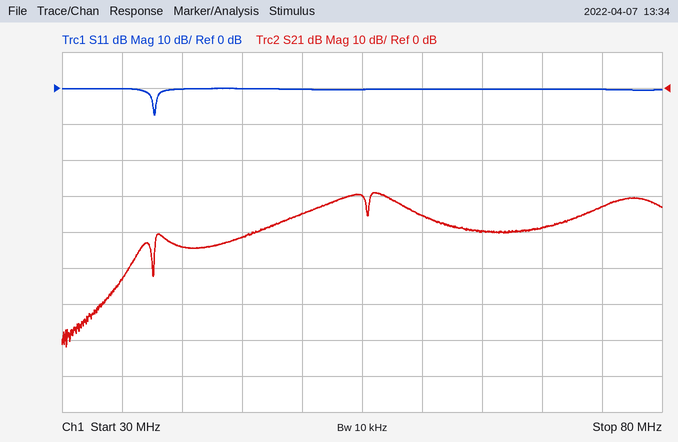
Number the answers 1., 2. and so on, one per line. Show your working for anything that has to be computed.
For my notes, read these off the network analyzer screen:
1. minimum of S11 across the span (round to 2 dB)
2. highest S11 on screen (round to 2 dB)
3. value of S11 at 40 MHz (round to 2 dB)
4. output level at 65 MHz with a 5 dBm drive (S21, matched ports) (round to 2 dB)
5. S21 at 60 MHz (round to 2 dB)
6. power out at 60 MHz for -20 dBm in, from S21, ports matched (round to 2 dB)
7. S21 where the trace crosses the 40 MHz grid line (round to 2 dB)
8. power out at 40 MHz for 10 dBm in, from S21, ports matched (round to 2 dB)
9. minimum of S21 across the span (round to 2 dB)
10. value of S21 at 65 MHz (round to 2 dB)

1. -8 dB
2. 0 dB
3. 0 dB
4. 5 dBm + (-40 dB) = -34 dBm
5. -36 dB
6. -20 dBm + (-36 dB) = -56 dBm
7. -44 dB
8. 10 dBm + (-44 dB) = -34 dBm
9. -72 dB
10. -40 dB
